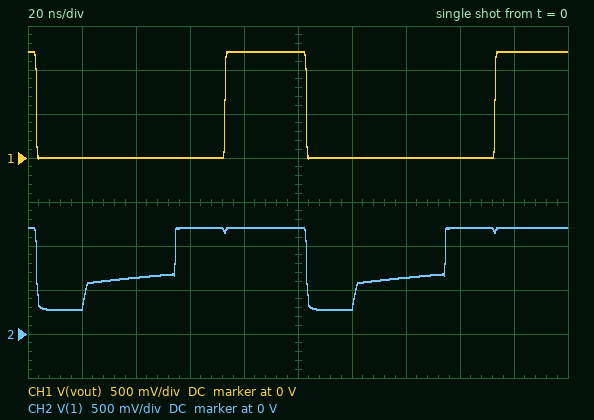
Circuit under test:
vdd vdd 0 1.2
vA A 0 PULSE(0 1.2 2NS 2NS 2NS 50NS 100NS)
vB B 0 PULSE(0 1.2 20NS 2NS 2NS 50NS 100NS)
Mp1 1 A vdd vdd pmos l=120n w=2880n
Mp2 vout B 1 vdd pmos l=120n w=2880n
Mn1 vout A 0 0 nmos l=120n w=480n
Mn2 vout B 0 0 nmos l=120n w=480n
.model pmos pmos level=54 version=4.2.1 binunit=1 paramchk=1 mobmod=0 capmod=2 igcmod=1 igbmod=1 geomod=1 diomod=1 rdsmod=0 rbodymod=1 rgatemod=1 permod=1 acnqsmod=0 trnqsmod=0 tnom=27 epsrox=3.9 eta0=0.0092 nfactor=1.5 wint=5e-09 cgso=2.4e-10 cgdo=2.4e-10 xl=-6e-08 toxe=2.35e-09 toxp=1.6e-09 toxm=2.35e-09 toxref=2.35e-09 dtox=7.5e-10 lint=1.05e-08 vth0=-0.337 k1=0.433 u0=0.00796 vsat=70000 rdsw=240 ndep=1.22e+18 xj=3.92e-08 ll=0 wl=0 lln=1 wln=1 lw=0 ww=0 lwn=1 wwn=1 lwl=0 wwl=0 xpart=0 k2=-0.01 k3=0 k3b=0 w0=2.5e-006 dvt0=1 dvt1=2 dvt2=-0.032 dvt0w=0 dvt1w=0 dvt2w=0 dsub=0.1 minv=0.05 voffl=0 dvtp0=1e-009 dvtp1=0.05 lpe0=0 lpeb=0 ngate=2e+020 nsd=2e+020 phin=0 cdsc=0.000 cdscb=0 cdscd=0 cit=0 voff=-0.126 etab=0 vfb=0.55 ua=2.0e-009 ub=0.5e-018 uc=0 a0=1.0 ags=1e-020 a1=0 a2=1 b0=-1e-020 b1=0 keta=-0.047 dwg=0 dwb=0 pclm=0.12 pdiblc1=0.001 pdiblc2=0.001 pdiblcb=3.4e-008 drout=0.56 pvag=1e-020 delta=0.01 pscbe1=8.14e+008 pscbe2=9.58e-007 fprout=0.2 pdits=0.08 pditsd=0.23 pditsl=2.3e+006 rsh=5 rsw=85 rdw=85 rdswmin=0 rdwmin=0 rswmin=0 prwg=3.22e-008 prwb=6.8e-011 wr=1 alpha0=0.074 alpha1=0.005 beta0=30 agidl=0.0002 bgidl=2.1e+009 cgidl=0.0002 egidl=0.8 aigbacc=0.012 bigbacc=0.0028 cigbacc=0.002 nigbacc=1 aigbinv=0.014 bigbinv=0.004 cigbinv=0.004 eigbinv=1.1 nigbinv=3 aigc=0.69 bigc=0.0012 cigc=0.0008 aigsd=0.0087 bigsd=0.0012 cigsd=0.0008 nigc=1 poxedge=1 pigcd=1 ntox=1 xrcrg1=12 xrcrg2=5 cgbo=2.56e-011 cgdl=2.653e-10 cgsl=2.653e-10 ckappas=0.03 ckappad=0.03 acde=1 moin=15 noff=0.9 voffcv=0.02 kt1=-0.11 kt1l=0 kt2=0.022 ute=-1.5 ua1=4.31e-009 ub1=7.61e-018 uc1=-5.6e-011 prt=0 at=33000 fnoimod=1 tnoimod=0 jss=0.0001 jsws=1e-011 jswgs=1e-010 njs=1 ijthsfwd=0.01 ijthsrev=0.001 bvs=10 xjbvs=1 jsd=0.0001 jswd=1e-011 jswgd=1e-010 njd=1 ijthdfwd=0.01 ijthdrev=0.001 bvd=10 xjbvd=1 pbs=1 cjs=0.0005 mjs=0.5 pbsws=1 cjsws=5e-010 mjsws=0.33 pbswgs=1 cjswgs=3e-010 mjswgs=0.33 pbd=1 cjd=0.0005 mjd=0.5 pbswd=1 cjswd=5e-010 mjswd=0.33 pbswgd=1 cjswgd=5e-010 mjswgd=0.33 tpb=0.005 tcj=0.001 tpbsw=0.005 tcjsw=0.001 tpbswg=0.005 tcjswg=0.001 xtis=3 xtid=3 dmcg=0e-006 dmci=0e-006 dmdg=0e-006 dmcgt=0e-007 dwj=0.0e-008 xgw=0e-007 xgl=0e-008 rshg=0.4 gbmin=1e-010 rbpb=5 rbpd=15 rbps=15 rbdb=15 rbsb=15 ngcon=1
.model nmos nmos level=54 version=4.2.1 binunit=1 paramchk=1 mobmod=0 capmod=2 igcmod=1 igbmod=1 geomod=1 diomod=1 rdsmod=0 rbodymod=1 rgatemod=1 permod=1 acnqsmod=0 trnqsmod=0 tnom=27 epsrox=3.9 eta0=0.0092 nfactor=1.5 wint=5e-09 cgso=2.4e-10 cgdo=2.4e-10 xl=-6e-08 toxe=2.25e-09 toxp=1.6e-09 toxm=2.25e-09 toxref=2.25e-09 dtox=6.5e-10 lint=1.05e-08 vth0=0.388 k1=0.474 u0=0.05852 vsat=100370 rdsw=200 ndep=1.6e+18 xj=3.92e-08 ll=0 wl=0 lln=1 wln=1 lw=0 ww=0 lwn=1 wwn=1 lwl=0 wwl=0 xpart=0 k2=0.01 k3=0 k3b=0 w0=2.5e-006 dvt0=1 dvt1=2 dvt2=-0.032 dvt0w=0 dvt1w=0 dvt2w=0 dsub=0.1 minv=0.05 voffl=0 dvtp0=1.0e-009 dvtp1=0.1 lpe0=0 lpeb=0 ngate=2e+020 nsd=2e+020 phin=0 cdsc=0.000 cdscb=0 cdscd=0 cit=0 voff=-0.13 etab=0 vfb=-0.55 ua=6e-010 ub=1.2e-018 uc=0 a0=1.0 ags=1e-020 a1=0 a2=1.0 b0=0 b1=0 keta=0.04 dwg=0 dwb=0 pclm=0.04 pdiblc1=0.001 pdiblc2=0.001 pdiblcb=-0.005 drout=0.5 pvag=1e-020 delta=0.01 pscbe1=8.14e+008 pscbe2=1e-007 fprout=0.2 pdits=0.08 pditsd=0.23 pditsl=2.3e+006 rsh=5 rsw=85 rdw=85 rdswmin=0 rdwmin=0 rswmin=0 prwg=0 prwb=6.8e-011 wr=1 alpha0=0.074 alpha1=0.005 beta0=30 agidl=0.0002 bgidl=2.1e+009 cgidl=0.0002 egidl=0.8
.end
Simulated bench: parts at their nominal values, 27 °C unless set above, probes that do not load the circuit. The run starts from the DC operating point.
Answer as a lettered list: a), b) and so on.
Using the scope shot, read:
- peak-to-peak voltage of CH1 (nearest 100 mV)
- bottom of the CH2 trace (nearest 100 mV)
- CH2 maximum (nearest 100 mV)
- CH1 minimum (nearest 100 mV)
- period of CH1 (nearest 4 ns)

a) 1.2 V
b) 300 mV
c) 1.2 V
d) 0 V
e) 100 ns
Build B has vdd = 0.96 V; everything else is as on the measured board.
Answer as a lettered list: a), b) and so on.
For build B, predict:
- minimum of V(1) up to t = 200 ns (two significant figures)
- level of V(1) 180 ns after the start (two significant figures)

a) 190 mV
b) 960 mV
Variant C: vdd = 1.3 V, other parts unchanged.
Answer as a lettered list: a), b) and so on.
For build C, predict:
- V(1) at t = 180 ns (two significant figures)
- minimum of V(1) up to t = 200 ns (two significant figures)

a) 1.3 V
b) 360 mV
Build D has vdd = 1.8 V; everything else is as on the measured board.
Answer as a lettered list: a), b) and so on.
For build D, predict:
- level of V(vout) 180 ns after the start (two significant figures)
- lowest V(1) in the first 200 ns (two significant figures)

a) 1.8 V
b) 870 mV
